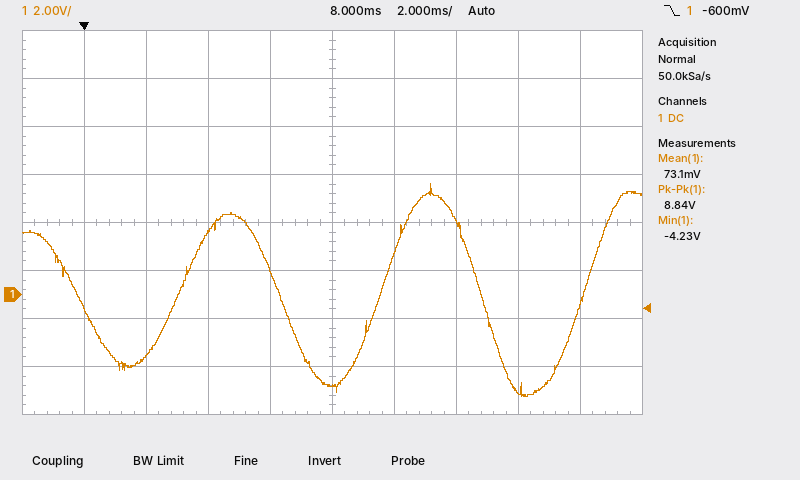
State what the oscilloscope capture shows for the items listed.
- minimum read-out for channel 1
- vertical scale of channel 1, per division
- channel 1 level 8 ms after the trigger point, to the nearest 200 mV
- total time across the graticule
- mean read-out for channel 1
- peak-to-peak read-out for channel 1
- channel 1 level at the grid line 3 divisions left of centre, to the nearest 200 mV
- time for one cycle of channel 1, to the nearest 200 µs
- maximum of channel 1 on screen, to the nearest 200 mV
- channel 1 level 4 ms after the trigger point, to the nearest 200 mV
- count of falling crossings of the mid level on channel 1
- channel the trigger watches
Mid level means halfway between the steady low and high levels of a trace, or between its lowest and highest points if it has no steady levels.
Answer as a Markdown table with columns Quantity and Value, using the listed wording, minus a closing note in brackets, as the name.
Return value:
| Quantity | Value |
|---|---|
| minimum read-out for channel 1 | -4.23 V |
| vertical scale of channel 1, per division | 2 V |
| channel 1 level 8 ms after the trigger point, to the nearest 200 mV | -3.8 V |
| total time across the graticule | 20 ms |
| mean read-out for channel 1 | 73.1 mV |
| peak-to-peak read-out for channel 1 | 8.84 V |
| channel 1 level at the grid line 3 divisions left of centre, to the nearest 200 mV | -2.6 V |
| time for one cycle of channel 1, to the nearest 200 µs | 6.6 ms |
| maximum of channel 1 on screen, to the nearest 200 mV | 4.6 V |
| channel 1 level 4 ms after the trigger point, to the nearest 200 mV | 2.6 V |
| count of falling crossings of the mid level on channel 1 | 3 |
| channel the trigger watches | channel 1 |
